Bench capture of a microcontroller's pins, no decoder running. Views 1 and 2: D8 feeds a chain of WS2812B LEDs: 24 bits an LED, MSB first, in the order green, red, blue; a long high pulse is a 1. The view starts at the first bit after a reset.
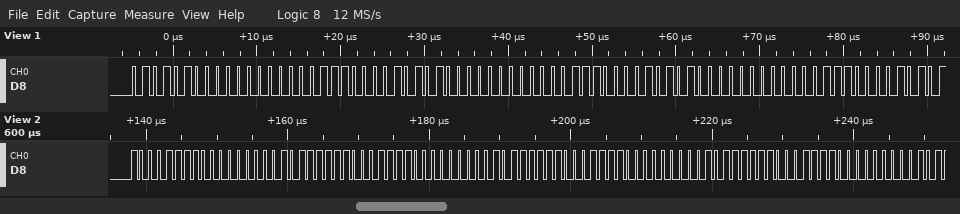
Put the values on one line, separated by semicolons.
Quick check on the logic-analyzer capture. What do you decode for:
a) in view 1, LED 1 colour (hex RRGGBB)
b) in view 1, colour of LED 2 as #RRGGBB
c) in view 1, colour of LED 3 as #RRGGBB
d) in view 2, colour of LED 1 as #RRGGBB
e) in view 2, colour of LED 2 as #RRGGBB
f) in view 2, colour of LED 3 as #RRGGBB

#005438; #005438; #005438; #008F5F; #008F5F; #008F5F
